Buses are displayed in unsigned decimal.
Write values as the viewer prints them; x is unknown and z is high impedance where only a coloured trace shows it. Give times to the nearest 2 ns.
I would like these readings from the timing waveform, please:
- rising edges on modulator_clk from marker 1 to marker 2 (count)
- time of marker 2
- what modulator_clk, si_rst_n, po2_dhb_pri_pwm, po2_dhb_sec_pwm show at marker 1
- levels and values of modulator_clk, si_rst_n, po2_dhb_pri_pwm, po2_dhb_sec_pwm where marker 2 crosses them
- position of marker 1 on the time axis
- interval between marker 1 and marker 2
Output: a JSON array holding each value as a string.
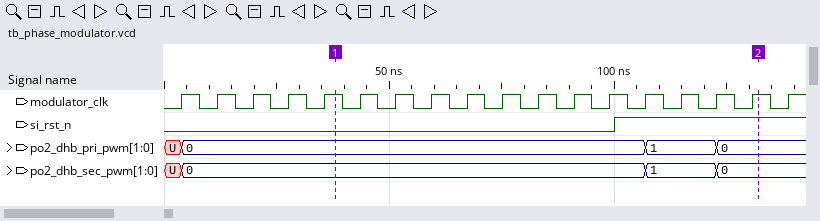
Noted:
["12", "132 ns", "modulator_clk=1, si_rst_n=0, po2_dhb_pri_pwm=0, po2_dhb_sec_pwm=0", "modulator_clk=1, si_rst_n=1, po2_dhb_pri_pwm=0, po2_dhb_sec_pwm=0", "38 ns", "94 ns"]
